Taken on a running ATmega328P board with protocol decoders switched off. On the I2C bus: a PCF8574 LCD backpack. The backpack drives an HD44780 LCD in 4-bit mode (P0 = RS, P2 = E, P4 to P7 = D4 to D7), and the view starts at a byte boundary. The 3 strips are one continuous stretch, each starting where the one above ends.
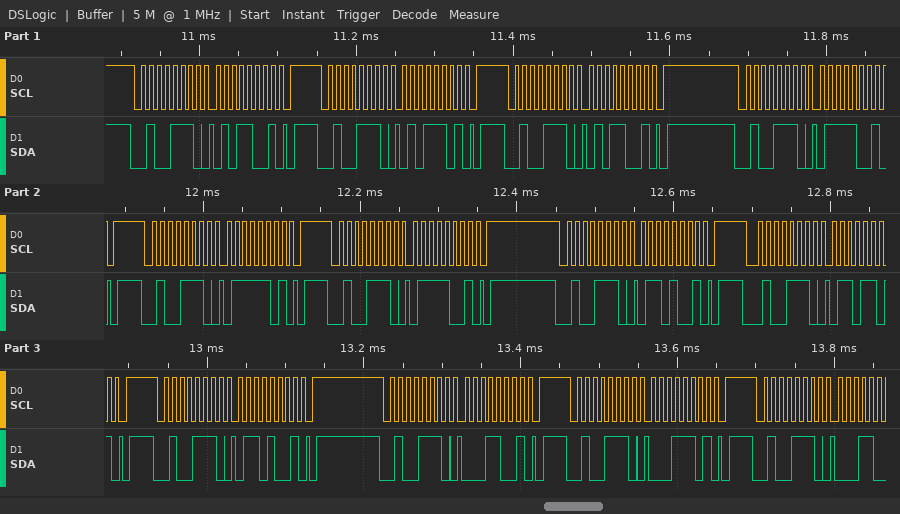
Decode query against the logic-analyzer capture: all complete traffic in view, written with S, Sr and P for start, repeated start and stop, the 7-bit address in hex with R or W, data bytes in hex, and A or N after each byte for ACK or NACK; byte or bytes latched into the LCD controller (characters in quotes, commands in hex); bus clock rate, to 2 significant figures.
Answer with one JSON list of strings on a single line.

["S 27W A 59 A P S 27W A 5D A P S 27W A 59 A P S 27W A 79 A P S 27W A 7D A P S 27W A 79 A P S 27W A 69 A P S 27W A 6D A P S 27W A 69 A P S 27W A 19 A P S 27W A 1D A P S 27W A", "'W'", "100 kHz"]
